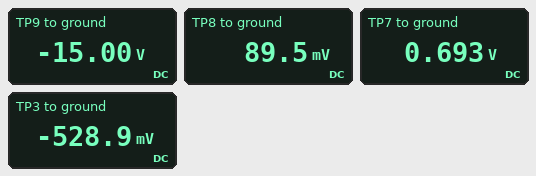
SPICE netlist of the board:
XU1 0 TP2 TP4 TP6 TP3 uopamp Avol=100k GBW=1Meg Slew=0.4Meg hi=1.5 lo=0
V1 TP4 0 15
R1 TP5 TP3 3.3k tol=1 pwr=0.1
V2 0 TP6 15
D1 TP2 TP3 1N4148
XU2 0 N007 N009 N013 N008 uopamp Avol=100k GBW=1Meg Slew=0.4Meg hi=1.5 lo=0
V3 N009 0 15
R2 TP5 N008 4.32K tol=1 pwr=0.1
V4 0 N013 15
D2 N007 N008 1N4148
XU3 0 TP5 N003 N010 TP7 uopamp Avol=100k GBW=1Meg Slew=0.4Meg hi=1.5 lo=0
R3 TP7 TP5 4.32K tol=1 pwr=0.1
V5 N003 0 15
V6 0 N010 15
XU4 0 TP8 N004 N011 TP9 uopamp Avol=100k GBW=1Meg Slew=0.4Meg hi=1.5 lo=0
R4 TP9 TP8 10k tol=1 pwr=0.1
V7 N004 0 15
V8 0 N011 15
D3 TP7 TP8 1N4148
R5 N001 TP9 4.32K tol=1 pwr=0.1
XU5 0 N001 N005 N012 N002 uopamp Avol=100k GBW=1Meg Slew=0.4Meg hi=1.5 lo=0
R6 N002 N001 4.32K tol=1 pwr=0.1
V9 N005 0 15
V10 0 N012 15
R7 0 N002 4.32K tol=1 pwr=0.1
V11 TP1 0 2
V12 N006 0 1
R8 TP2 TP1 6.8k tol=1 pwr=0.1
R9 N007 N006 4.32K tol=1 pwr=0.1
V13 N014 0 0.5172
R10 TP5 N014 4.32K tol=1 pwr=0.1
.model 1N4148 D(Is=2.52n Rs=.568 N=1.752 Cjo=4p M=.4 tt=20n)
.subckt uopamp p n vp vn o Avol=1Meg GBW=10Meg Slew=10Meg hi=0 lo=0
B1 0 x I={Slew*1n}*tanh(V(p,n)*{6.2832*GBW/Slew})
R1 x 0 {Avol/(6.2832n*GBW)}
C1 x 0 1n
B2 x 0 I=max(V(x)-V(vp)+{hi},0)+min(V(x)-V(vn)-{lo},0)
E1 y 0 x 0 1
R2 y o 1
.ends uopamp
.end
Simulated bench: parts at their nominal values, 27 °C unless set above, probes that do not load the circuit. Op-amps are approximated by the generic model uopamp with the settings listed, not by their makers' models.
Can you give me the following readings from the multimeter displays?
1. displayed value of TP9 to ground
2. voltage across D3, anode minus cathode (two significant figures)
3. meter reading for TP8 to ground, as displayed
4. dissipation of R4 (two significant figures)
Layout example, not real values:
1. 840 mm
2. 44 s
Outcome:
1. -15.00 V
2. 600 mV
3. 89.5 mV
4. 23 mW
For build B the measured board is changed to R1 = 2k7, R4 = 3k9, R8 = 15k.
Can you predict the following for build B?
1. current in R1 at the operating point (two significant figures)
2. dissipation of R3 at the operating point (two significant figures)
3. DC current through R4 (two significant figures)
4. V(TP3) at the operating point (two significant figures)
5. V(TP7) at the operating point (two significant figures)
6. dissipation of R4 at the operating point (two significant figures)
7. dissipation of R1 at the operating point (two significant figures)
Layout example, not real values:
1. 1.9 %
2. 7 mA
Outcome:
1. 180 µA
2. 140 µW
3. 3.9 mA
4. -490 mV
5. 790 mV
6. 59 mW
7. 90 µW
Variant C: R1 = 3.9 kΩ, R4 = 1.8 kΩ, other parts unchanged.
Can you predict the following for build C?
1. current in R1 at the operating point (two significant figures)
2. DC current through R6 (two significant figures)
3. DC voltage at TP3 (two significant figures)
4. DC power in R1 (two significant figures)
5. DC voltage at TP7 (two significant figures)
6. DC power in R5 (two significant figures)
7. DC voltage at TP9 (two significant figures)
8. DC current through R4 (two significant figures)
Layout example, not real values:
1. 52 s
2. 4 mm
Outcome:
1. 140 µA
2. 430 µA
3. -530 mV
4. 72 µW
5. 590 mV
6. 810 µW
7. -1.9 V
8. 1.0 mA
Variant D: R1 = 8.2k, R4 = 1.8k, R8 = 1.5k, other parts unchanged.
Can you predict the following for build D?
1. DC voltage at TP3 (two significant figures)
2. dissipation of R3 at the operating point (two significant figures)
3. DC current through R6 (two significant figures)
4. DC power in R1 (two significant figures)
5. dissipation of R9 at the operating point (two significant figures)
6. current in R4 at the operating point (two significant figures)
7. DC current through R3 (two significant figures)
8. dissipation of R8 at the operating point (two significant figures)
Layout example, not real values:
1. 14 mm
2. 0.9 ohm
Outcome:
1. -600 mV
2. 23 µW
3. 1.1 µA
4. 44 µW
5. 230 µW
6. 2.7 µA
7. 73 µA
8. 2.7 mW
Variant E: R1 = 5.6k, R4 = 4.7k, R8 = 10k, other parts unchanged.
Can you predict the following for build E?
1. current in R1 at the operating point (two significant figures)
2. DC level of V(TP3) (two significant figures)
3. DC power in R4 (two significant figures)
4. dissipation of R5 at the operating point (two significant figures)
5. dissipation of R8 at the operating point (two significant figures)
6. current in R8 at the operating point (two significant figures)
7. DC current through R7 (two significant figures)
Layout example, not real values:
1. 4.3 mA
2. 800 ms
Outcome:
1. 91 µA
2. -510 mV
3. 1.1 µW
4. 1.2 µW
5. 400 µW
6. 200 µA
7. 17 µA
